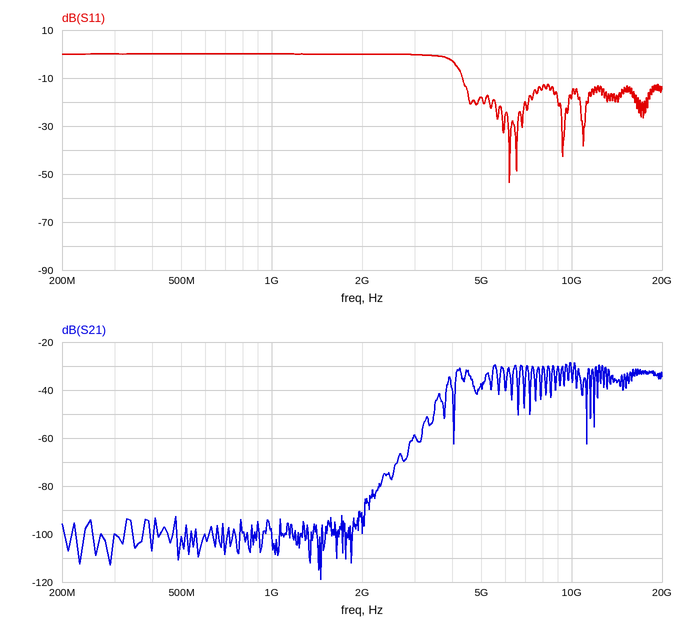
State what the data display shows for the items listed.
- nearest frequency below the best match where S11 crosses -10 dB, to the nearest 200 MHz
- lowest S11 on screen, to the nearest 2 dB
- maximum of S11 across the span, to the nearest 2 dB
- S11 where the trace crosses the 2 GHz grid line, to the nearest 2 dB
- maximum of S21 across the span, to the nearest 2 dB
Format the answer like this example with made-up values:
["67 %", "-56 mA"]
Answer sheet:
["4.4 GHz", "-54 dB", "0 dB", "0 dB", "-28 dB"]
